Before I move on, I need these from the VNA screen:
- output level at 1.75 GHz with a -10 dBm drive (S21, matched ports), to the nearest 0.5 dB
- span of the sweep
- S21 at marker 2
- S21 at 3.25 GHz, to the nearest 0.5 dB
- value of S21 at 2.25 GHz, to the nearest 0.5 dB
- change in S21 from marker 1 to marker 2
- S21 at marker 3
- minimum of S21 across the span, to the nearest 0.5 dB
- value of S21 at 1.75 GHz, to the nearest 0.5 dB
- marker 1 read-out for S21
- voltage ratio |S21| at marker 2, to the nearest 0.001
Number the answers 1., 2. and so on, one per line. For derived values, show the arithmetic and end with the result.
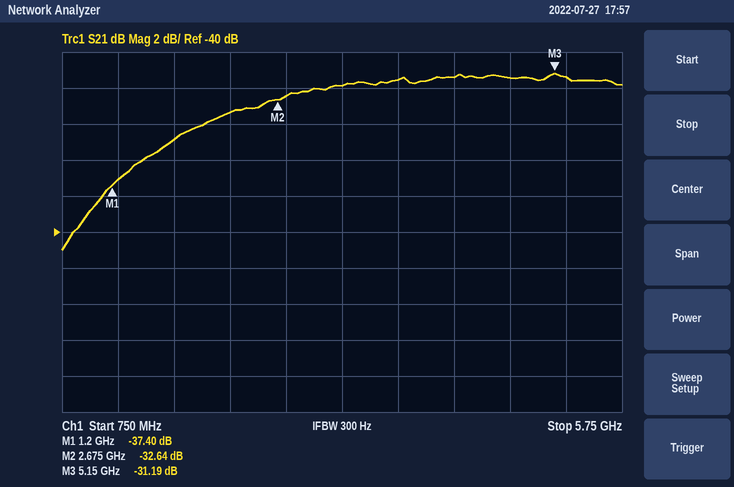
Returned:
1. -10 dBm + (-35.0 dB) = -45.0 dBm
2. 5 GHz
3. -32.64 dB
4. -32.0 dB
5. -33.5 dB
6. -32.64 − (-37.4) = 4.76 dB
7. -31.19 dB
8. -41.0 dB
9. -35.0 dB
10. -37.40 dB
11. 10^(-32.64/20) ≈ 0.023
